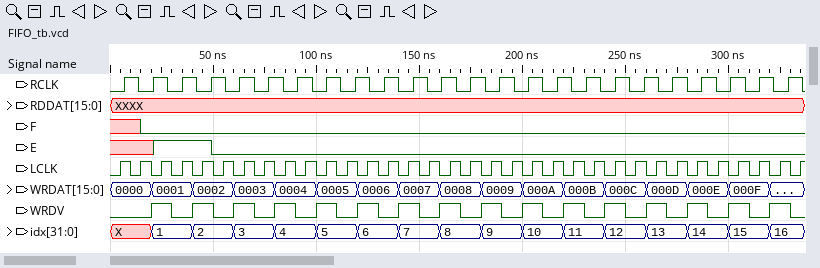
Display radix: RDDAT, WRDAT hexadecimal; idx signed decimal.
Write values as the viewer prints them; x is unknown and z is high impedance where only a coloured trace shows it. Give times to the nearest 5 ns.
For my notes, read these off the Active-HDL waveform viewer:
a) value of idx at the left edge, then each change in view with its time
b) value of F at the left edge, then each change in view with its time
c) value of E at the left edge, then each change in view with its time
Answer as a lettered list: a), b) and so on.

a) X, 1 at 20 ns, 2 at 40 ns, 3 at 60 ns, 4 at 80 ns, 5 at 100 ns, 6 at 120 ns, 7 at 140 ns, 8 at 160 ns, 9 at 180 ns, 10 at 200 ns, 11 at 220 ns, 12 at 240 ns, 13 at 260 ns, 14 at 280 ns, 15 at 300 ns, 16 at 320 ns
b) x, 0 at 15 ns
c) x, 1 at 20 ns, 0 at 50 ns
